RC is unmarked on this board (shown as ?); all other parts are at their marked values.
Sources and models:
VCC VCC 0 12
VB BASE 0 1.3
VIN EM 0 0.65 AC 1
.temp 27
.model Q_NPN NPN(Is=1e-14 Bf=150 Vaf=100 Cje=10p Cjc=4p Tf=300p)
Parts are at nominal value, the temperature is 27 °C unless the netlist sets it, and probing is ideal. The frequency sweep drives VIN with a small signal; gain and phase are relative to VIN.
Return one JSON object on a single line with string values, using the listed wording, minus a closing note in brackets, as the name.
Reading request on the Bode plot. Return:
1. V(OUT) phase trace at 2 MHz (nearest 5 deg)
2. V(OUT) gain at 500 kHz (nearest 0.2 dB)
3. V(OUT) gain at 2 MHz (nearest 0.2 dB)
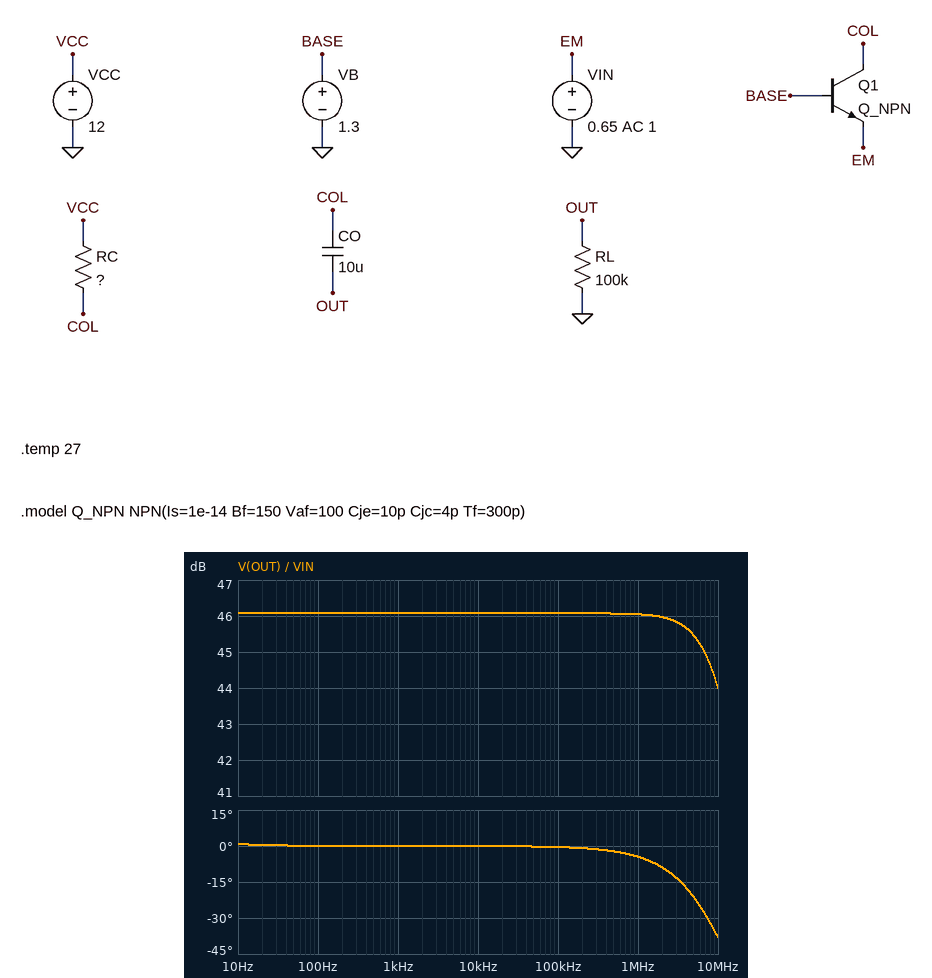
{"V(OUT) phase trace at 2 MHz": "-10 deg", "V(OUT) gain at 500 kHz": "46.0 dB", "V(OUT) gain at 2 MHz": "46.0 dB"}
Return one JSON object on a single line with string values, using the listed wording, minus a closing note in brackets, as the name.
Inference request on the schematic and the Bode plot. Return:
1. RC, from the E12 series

{"RC, from the E12 series": "6.8 kΩ"}
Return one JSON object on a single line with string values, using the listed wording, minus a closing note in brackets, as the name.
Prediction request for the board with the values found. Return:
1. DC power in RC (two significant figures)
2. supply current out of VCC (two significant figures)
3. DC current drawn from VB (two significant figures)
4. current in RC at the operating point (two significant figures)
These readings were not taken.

{"DC power in RC": "5.0 mW", "supply current out of VCC": "860 µA", "DC current drawn from VB": "5.5 µA", "current in RC at the operating point": "860 µA"}
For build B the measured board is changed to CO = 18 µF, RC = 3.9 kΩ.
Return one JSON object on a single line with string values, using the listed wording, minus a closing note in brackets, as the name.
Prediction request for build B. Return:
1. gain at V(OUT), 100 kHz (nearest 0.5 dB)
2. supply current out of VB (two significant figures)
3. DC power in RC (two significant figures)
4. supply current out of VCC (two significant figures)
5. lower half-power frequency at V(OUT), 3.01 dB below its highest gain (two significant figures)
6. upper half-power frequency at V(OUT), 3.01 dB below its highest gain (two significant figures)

{"gain at V(OUT), 100 kHz": "42.0 dB", "supply current out of VB": "5.5 µA", "DC power in RC": "3.0 mW", "supply current out of VCC": "880 µA", "lower half-power frequency at V(OUT), 3.01 dB below its highest gain": "85 mHz", "upper half-power frequency at V(OUT), 3.01 dB below its highest gain": "24 MHz"}
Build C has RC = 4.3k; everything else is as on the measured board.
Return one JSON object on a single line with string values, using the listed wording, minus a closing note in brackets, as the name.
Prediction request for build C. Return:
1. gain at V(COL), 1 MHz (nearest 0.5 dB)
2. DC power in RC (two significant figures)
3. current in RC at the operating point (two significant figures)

{"gain at V(COL), 1 MHz": "42.5 dB", "DC power in RC": "3.3 mW", "current in RC at the operating point": "880 µA"}
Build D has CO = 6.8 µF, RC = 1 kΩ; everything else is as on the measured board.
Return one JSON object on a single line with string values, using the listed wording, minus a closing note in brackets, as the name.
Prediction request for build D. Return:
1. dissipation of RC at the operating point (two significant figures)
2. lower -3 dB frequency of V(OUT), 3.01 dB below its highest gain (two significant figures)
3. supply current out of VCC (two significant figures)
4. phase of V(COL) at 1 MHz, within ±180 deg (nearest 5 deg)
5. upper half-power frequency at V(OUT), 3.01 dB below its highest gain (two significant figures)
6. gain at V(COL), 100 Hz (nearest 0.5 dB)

{"dissipation of RC at the operating point": "810 µW", "lower -3 dB frequency of V(OUT), 3.01 dB below its highest gain": "230 mHz", "supply current out of VCC": "900 µA", "phase of V(COL) at 1 MHz, within ±180 deg": "0 deg", "upper half-power frequency at V(OUT), 3.01 dB below its highest gain": "97 MHz", "gain at V(COL), 100 Hz": "30.5 dB"}
